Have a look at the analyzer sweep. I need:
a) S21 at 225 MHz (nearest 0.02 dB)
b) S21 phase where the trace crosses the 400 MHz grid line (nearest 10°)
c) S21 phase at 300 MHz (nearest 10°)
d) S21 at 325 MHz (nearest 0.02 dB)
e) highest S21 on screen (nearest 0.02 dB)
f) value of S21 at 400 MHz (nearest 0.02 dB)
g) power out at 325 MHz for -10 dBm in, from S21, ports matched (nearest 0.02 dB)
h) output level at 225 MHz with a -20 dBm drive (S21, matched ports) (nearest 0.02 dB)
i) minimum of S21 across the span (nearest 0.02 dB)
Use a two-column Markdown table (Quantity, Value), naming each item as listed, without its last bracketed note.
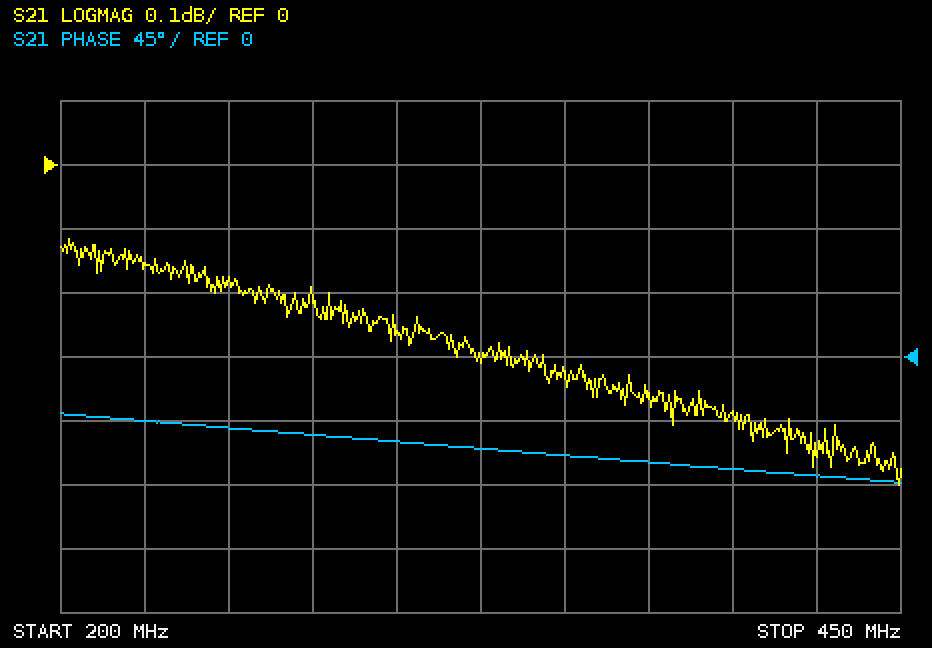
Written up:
| Quantity | Value |
|---|---|
| S21 at 225 MHz | -0.16 dB |
| S21 phase where the trace crosses the 400 MHz grid line | -80° |
| S21 phase at 300 MHz | -60° |
| S21 at 325 MHz | -0.30 dB |
| highest S21 on screen | -0.12 dB |
| value of S21 at 400 MHz | -0.38 dB |
| power out at 325 MHz for -10 dBm in, from S21, ports matched | -10.30 dBm |
| output level at 225 MHz with a -20 dBm drive (S21, matched ports) | -20.16 dBm |
| minimum of S21 across the span | -0.50 dB |
